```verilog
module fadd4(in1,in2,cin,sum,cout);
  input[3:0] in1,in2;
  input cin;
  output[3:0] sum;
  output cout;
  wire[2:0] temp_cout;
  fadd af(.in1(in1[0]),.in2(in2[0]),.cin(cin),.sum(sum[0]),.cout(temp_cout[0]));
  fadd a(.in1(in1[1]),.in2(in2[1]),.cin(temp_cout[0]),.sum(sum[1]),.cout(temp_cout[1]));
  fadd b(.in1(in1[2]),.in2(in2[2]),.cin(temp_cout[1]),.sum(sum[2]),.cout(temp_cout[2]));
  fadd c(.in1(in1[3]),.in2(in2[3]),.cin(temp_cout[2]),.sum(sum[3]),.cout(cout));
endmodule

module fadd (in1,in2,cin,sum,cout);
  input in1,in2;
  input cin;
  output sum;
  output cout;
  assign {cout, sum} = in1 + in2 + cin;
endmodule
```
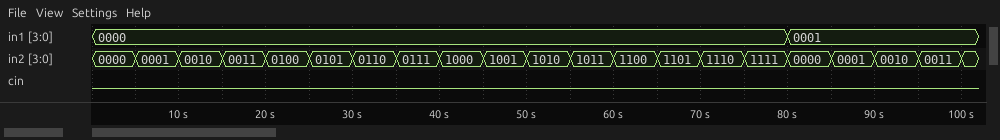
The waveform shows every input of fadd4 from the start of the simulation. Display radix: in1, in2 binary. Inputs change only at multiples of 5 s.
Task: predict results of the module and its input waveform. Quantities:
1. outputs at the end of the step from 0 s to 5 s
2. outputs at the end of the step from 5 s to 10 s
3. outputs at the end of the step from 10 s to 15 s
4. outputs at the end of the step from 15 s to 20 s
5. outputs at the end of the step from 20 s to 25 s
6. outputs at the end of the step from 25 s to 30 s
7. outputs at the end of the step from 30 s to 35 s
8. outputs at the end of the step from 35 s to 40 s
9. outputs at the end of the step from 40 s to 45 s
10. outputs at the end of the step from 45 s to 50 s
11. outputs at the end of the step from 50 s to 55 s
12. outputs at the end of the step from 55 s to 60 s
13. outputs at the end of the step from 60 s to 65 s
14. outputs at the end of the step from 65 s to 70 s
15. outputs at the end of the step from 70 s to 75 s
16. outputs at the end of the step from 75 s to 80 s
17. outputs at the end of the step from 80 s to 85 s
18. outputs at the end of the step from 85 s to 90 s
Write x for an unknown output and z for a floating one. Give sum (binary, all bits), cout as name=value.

sum=0000, cout=0
sum=0001, cout=0
sum=0010, cout=0
sum=0011, cout=0
sum=0100, cout=0
sum=0101, cout=0
sum=0110, cout=0
sum=0111, cout=0
sum=1000, cout=0
sum=1001, cout=0
sum=1010, cout=0
sum=1011, cout=0
sum=1100, cout=0
sum=1101, cout=0
sum=1110, cout=0
sum=1111, cout=0
sum=0001, cout=0
sum=0010, cout=0
